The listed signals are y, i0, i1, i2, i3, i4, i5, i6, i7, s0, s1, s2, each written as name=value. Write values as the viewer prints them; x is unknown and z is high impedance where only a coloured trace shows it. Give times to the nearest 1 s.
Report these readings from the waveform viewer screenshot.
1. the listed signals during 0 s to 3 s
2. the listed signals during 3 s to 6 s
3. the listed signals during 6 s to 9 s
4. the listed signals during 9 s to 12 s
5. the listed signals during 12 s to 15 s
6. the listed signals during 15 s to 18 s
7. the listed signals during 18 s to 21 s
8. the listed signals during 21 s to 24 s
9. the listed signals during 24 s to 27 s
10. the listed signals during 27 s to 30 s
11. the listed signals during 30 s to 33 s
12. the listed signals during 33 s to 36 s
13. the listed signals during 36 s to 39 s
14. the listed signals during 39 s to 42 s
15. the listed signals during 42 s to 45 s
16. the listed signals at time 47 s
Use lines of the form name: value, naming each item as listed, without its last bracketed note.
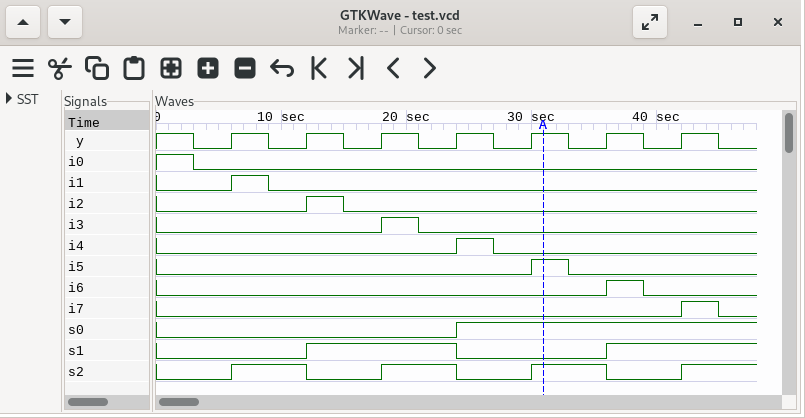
the listed signals during 0 s to 3 s: y=1, i0=1, i1=0, i2=0, i3=0, i4=0, i5=0, i6=0, i7=0, s0=0, s1=0, s2=0
the listed signals during 3 s to 6 s: y=0, i0=0, i1=0, i2=0, i3=0, i4=0, i5=0, i6=0, i7=0, s0=0, s1=0, s2=0
the listed signals during 6 s to 9 s: y=1, i0=0, i1=1, i2=0, i3=0, i4=0, i5=0, i6=0, i7=0, s0=0, s1=0, s2=1
the listed signals during 9 s to 12 s: y=0, i0=0, i1=0, i2=0, i3=0, i4=0, i5=0, i6=0, i7=0, s0=0, s1=0, s2=1
the listed signals during 12 s to 15 s: y=1, i0=0, i1=0, i2=1, i3=0, i4=0, i5=0, i6=0, i7=0, s0=0, s1=1, s2=0
the listed signals during 15 s to 18 s: y=0, i0=0, i1=0, i2=0, i3=0, i4=0, i5=0, i6=0, i7=0, s0=0, s1=1, s2=0
the listed signals during 18 s to 21 s: y=1, i0=0, i1=0, i2=0, i3=1, i4=0, i5=0, i6=0, i7=0, s0=0, s1=1, s2=1
the listed signals during 21 s to 24 s: y=0, i0=0, i1=0, i2=0, i3=0, i4=0, i5=0, i6=0, i7=0, s0=0, s1=1, s2=1
the listed signals during 24 s to 27 s: y=1, i0=0, i1=0, i2=0, i3=0, i4=1, i5=0, i6=0, i7=0, s0=1, s1=0, s2=0
the listed signals during 27 s to 30 s: y=0, i0=0, i1=0, i2=0, i3=0, i4=0, i5=0, i6=0, i7=0, s0=1, s1=0, s2=0
the listed signals during 30 s to 33 s: y=1, i0=0, i1=0, i2=0, i3=0, i4=0, i5=1, i6=0, i7=0, s0=1, s1=0, s2=1
the listed signals during 33 s to 36 s: y=0, i0=0, i1=0, i2=0, i3=0, i4=0, i5=0, i6=0, i7=0, s0=1, s1=0, s2=1
the listed signals during 36 s to 39 s: y=1, i0=0, i1=0, i2=0, i3=0, i4=0, i5=0, i6=1, i7=0, s0=1, s1=1, s2=0
the listed signals during 39 s to 42 s: y=0, i0=0, i1=0, i2=0, i3=0, i4=0, i5=0, i6=0, i7=0, s0=1, s1=1, s2=0
the listed signals during 42 s to 45 s: y=1, i0=0, i1=0, i2=0, i3=0, i4=0, i5=0, i6=0, i7=1, s0=1, s1=1, s2=1
the listed signals at time 47 s: y=0, i0=0, i1=0, i2=0, i3=0, i4=0, i5=0, i6=0, i7=0, s0=1, s1=1, s2=1
